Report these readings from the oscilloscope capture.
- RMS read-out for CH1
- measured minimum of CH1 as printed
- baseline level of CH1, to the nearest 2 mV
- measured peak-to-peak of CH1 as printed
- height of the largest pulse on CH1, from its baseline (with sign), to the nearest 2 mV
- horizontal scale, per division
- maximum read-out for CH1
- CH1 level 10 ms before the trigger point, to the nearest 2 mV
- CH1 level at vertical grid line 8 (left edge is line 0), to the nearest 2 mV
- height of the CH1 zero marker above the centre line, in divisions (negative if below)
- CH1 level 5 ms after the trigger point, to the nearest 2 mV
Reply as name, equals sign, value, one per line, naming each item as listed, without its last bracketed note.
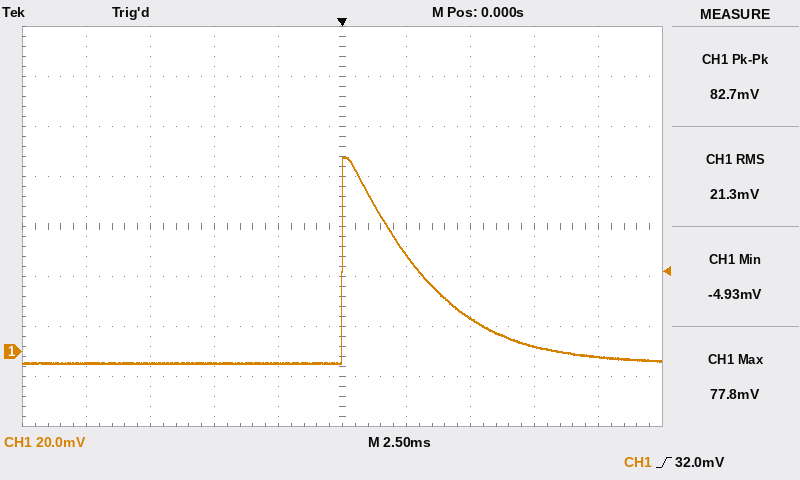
RMS read-out for CH1 = 21.3 mV
measured minimum of CH1 as printed = -4.93 mV
baseline level of CH1, to the nearest 2 mV = -4 mV
measured peak-to-peak of CH1 as printed = 82.7 mV
height of the largest pulse on CH1, from its baseline (with sign), to the nearest 2 mV = +82 mV
horizontal scale, per division = 2.5 ms
maximum read-out for CH1 = 77.8 mV
CH1 level 10 ms before the trigger point, to the nearest 2 mV = -4 mV
CH1 level at vertical grid line 8 (left edge is line 0), to the nearest 2 mV = 2 mV
height of the CH1 zero marker above the centre line, in divisions = -2.5 div
CH1 level 5 ms after the trigger point, to the nearest 2 mV = 14 mV
